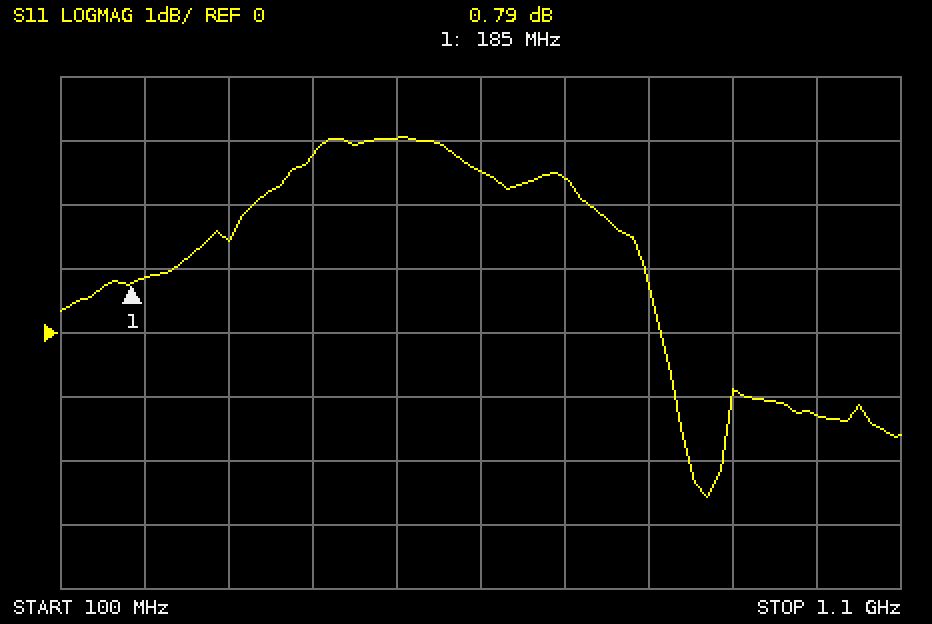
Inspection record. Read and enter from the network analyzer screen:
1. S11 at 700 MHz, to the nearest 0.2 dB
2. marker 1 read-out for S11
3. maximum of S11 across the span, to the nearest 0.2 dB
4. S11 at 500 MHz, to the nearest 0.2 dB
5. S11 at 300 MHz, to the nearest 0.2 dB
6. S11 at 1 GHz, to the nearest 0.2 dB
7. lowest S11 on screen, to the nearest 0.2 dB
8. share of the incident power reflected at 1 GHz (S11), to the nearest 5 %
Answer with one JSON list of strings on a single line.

["2.4 dB", "0.79 dB", "3.0 dB", "3.0 dB", "1.4 dB", "-1.2 dB", "-2.6 dB", "75 %"]
